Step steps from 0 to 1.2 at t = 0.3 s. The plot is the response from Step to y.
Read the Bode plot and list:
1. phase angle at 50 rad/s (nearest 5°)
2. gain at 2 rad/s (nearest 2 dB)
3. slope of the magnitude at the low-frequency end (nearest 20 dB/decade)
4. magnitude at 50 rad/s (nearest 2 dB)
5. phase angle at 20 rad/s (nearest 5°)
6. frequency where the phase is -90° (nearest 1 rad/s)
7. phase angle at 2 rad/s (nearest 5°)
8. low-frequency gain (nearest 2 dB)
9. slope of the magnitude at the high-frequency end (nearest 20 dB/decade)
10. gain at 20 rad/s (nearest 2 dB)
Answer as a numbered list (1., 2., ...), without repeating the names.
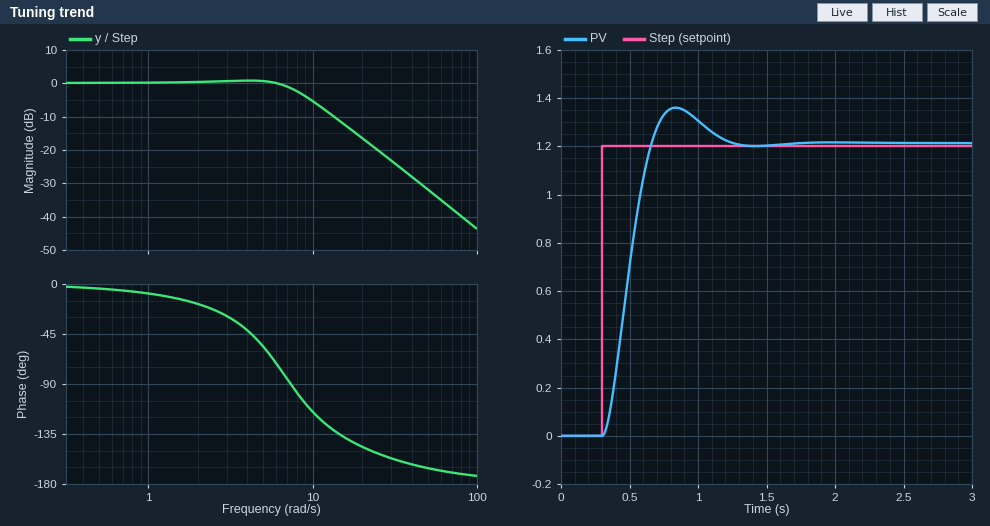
1. -165°
2. 0 dB
3. 0 dB/decade
4. -32 dB
5. -145°
6. 7 rad/s
7. -20°
8. 0 dB
9. -40 dB/decade
10. -16 dB
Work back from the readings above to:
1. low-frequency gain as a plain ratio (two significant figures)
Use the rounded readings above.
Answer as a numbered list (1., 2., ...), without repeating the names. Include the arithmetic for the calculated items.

1. 10^(0 / 20) = 1.0
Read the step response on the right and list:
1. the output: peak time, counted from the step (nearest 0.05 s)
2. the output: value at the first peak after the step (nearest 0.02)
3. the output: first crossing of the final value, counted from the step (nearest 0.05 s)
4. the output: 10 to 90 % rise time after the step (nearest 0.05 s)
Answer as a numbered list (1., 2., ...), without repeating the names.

1. 0.55 s
2. 1.36
3. 0.35 s
4. 0.25 s
